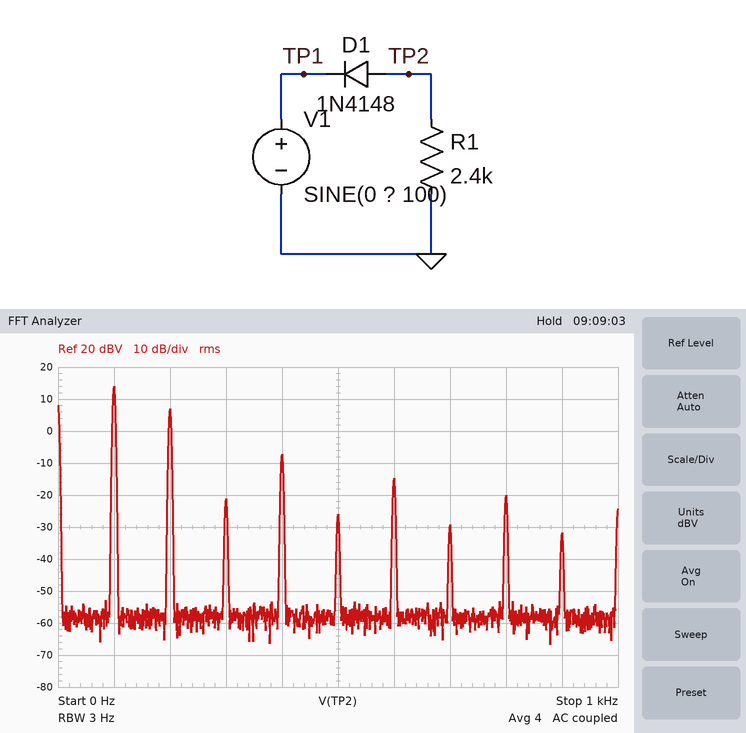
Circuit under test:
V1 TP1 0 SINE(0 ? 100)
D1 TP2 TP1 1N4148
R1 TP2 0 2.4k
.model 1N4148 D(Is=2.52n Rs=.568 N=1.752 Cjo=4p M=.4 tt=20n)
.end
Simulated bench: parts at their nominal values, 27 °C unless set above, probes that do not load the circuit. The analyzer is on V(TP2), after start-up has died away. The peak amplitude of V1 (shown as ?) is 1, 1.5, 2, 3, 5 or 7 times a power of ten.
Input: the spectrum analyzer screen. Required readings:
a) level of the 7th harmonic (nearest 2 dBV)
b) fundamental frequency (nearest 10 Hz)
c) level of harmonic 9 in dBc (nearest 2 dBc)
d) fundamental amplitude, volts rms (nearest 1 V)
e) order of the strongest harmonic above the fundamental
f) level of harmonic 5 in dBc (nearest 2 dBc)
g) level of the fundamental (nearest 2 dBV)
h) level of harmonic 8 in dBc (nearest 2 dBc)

-30 dBV
100 Hz
-46 dBc
5 V
2
-40 dBc
14 dBV
-34 dBc
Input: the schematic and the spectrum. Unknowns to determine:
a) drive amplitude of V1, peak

15 V
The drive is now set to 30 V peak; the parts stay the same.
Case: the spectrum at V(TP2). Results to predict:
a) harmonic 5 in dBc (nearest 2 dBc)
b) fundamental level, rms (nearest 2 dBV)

-46 dBc
20 dBV
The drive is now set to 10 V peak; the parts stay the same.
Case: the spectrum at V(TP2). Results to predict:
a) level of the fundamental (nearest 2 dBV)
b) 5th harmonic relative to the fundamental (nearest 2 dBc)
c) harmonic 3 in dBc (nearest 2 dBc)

10 dBV
-36 dBc
-32 dBc
